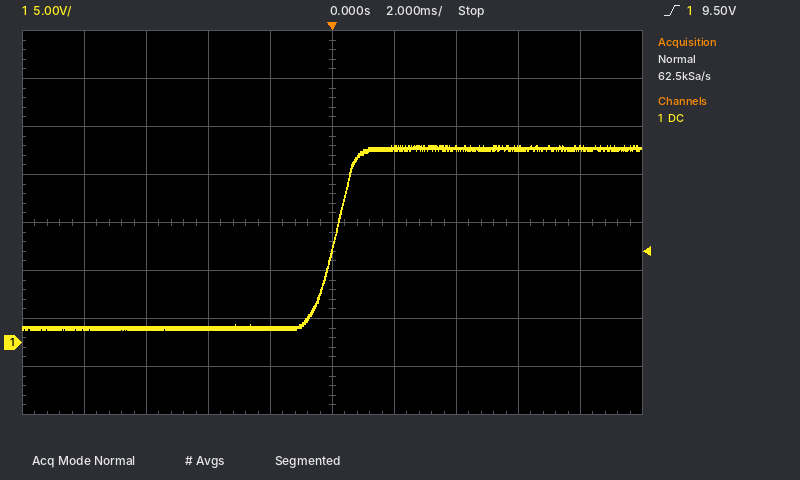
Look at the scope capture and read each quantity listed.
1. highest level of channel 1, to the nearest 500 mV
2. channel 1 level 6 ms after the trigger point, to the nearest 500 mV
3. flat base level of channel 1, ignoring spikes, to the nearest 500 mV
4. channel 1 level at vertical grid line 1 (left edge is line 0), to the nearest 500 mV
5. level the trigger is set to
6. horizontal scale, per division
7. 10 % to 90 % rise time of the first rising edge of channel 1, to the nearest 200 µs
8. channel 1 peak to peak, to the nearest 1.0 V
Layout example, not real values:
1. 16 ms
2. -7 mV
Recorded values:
1. 20.5 V
2. 20.0 V
3. 1.5 V
4. 1.5 V
5. 9.50 V
6. 2 ms
7. 1.2 ms
8. 19.0 V
